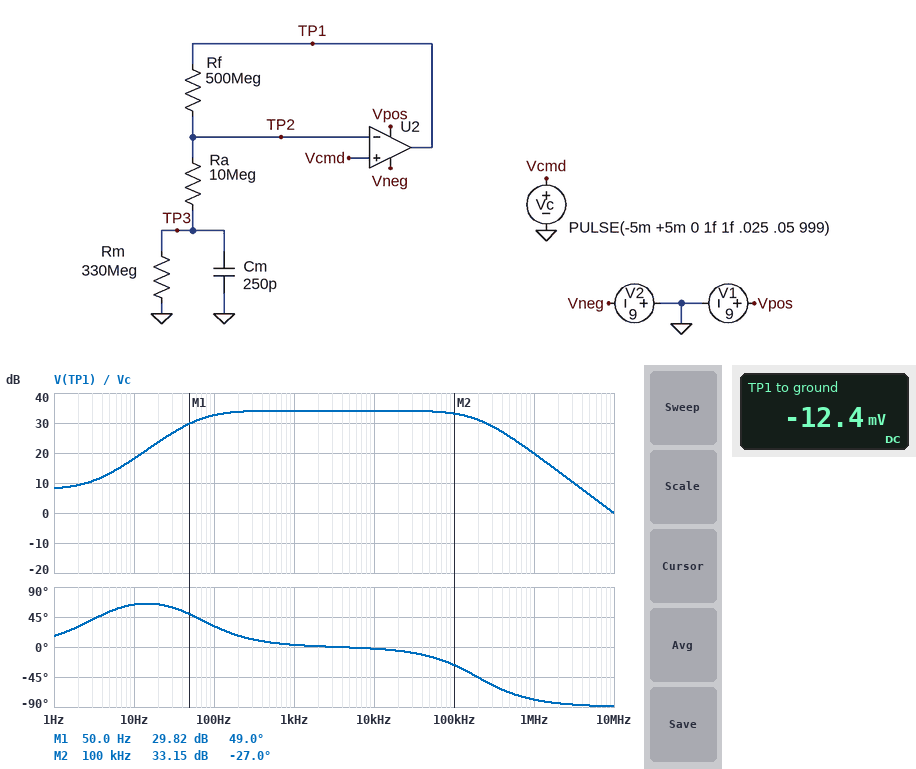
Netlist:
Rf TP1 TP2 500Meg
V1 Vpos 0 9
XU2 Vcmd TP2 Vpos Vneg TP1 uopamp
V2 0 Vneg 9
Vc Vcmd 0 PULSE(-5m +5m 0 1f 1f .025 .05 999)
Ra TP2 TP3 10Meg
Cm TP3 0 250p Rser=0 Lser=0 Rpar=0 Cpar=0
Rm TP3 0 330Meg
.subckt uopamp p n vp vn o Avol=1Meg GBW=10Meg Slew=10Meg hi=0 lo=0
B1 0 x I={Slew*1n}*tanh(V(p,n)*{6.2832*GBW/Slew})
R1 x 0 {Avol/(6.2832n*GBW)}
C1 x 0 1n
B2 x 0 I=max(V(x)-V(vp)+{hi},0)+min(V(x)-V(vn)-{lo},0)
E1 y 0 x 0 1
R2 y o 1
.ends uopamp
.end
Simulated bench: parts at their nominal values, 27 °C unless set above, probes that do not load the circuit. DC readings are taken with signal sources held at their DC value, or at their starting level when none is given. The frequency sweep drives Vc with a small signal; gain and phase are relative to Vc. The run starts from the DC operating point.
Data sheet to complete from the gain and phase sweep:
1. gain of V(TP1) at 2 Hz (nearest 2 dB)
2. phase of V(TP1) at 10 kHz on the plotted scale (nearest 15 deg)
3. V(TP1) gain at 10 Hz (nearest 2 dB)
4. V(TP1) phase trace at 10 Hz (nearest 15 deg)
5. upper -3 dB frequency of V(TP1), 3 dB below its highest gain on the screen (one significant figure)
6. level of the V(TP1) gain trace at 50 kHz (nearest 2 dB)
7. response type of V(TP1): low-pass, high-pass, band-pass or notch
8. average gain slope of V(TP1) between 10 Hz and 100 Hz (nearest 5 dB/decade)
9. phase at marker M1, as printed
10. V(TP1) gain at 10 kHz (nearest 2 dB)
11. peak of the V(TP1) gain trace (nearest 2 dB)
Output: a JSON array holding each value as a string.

["10 dB", "0 deg", "18 dB", "60 deg", "200 kHz", "34 dB", "band-pass", "15 dB/decade", "49.0 deg", "34 dB", "34 dB"]
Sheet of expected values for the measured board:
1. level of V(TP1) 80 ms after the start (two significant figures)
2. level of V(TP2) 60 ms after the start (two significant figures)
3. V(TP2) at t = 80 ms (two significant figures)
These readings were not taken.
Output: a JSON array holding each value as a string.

["-74 mV", "5.0 mV", "-5.0 mV"]
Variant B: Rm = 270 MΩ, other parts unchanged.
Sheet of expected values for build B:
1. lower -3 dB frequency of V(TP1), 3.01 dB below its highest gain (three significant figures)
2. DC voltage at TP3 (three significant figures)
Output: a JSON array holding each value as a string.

["65.8 Hz", "-4.82 mV"]
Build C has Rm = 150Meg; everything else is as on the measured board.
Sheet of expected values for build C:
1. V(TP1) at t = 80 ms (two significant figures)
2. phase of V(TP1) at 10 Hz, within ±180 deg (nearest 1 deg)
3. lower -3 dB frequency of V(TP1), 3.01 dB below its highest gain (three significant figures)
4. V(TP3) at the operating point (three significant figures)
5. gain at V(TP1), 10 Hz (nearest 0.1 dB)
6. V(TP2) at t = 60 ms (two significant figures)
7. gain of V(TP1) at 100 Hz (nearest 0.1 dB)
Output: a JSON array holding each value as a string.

["-76 mV", "53 deg", "67.4 Hz", "-4.69 mV", "18.6 dB", "5.0 mV", "32.5 dB"]
